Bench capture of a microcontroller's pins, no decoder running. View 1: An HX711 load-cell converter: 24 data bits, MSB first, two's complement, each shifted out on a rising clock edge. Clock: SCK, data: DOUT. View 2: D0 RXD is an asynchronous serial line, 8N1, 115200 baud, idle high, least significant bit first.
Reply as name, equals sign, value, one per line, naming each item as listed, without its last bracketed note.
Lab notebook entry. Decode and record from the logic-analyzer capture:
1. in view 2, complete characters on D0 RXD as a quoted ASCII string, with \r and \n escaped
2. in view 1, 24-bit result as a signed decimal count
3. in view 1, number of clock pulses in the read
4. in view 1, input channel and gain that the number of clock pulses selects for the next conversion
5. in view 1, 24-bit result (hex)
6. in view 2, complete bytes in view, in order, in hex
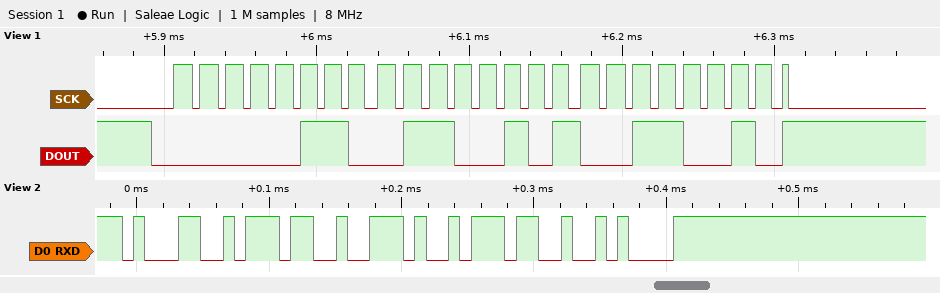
in view 2, complete characters on D0 RXD as a quoted ASCII string, with \r and \n escaped = "17.7\n"
in view 1, 24-bit result as a signed decimal count = 419122
in view 1, number of clock pulses in the read = 25
in view 1, input channel and gain that the number of clock pulses selects for the next conversion = channel A, gain 128
in view 1, 24-bit result = 0x066532
in view 2, complete bytes in view, in order, in hex = 0x31 0x37 0x2E 0x37 0x0A
